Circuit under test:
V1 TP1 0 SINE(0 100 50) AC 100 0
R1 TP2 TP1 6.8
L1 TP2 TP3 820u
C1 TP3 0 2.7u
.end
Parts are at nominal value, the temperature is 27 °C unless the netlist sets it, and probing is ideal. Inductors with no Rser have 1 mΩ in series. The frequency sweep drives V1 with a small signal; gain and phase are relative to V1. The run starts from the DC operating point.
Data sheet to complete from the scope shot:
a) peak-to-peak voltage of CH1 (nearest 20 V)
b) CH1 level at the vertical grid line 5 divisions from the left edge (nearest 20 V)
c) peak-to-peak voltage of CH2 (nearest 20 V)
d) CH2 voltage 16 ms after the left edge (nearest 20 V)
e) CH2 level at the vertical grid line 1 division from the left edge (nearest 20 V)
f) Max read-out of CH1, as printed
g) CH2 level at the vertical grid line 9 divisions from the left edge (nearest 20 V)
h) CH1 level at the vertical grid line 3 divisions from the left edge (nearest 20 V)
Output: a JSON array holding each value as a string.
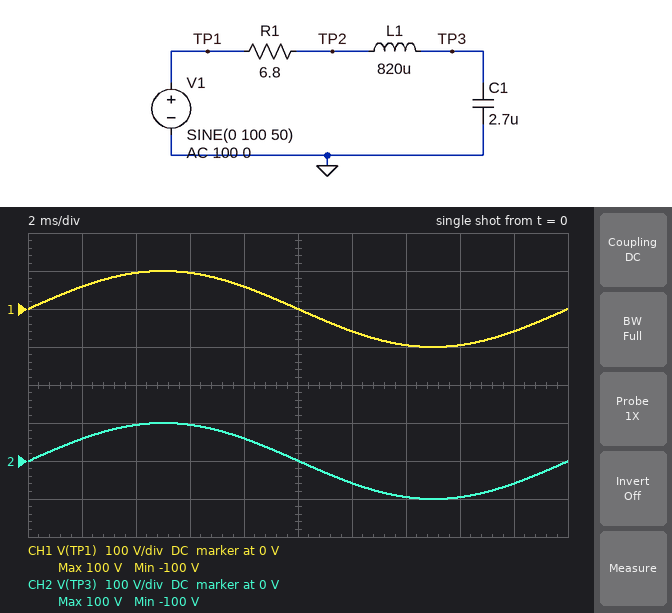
["200 V", "0 V", "200 V", "-100 V", "60 V", "100 V", "-60 V", "100 V"]
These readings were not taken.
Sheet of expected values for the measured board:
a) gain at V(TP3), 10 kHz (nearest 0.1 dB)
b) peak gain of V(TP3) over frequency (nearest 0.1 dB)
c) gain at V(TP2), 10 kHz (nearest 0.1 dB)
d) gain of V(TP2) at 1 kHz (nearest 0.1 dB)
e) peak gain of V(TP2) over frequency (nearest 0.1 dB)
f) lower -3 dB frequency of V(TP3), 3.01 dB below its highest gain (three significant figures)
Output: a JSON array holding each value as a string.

["-17.9 dB", "8.3 dB", "-0.1 dB", "-0.1 dB", "0 dB", "2.49 kHz"]
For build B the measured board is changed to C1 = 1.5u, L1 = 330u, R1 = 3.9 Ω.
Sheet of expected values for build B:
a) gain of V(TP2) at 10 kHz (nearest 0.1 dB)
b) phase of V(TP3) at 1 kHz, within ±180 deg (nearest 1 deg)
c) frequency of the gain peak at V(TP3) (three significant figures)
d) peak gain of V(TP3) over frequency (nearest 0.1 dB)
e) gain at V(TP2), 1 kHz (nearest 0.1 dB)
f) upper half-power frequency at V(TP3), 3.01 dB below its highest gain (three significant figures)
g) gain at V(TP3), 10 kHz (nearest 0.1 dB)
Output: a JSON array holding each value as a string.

["-0.6 dB", "-2 deg", "7.03 kHz", "11.7 dB", "0 dB", "7.92 kHz", "-0.2 dB"]
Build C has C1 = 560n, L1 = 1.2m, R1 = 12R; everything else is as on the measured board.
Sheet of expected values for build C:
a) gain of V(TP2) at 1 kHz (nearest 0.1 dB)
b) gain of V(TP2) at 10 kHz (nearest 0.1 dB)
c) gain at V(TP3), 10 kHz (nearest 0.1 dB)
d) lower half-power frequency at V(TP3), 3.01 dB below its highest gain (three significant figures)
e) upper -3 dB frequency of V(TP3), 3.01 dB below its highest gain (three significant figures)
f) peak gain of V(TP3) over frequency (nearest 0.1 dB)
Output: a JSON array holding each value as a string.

["0 dB", "-0.3 dB", "-4.6 dB", "5.17 kHz", "6.79 kHz", "11.8 dB"]
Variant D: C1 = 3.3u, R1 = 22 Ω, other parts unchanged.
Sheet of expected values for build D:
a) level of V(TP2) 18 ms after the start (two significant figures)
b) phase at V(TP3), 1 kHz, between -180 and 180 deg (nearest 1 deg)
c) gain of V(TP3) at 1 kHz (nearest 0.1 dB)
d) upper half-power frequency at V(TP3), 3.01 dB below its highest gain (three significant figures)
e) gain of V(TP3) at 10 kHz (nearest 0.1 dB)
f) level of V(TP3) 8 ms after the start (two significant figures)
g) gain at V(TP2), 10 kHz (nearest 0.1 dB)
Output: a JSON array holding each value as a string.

["-61 V", "-27 deg", "0 dB", "3.10 kHz", "-20.6 dB", "61 V", "-0.9 dB"]
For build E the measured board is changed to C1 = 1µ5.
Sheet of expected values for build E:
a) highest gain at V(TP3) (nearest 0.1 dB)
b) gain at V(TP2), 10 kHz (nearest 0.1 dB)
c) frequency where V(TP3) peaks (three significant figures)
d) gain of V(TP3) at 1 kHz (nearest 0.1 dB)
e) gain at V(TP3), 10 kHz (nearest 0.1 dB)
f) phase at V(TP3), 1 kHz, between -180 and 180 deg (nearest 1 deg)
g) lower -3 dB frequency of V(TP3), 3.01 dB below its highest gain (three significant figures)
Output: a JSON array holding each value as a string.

["10.8 dB", "-0.1 dB", "4.44 kHz", "0.4 dB", "-11.8 dB", "-4 deg", "3.71 kHz"]
